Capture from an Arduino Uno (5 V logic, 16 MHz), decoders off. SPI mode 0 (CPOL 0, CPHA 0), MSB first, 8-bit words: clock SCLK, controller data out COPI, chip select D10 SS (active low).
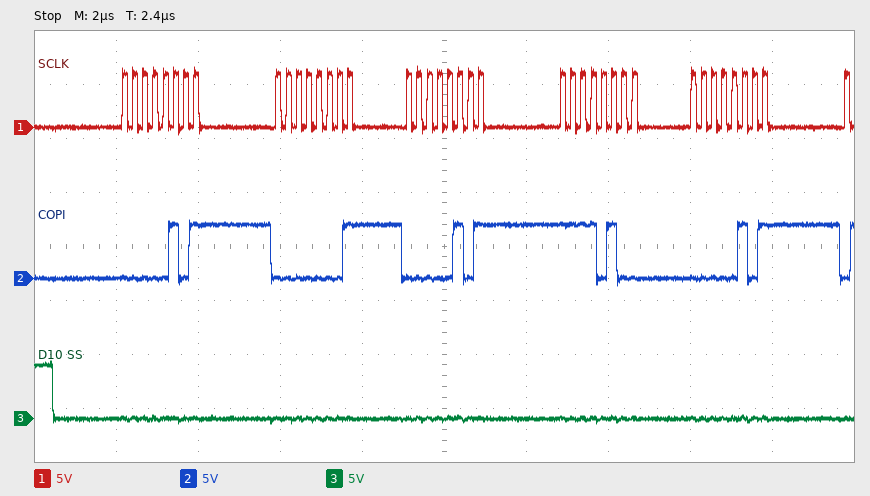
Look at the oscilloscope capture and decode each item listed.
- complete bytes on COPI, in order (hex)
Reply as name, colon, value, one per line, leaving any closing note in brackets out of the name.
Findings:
complete bytes on COPI, in order: 0x05 0x01 0x05 0xF4 0x05
